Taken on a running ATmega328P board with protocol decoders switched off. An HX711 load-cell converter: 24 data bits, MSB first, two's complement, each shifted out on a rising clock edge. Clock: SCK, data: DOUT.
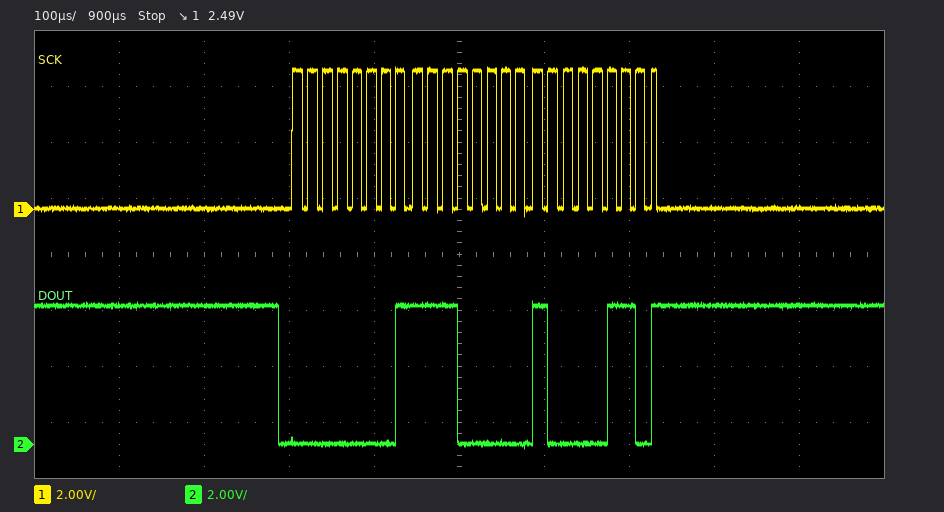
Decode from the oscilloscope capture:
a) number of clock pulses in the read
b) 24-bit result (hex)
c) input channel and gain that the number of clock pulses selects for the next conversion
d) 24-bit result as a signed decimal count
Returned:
25
0x01E086
channel A, gain 128
123014
